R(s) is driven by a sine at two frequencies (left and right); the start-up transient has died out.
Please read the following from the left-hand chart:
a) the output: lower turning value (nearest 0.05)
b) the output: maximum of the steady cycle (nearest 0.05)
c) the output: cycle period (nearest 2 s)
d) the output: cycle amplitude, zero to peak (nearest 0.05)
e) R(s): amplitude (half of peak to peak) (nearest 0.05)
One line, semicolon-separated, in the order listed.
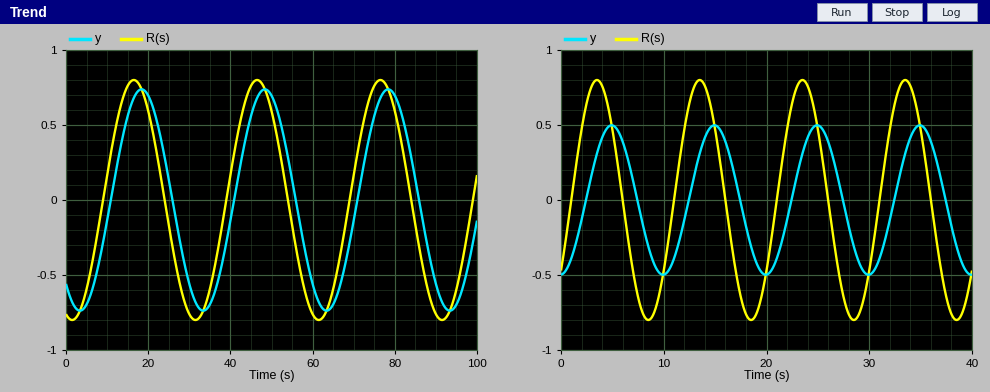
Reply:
-0.75; 0.75; 30 s; 0.75; 0.80
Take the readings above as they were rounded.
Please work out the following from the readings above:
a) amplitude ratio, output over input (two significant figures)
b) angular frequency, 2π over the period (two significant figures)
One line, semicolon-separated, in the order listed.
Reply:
0.94; 0.21 rad/s
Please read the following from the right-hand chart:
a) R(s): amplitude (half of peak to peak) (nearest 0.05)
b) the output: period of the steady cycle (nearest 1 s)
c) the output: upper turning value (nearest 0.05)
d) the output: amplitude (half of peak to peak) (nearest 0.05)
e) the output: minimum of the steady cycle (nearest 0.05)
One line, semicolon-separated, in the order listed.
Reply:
0.80; 10 s; 0.50; 0.50; -0.50
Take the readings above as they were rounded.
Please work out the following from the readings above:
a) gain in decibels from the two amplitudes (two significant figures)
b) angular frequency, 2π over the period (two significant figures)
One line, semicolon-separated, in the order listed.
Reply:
-4.1 dB; 0.63 rad/s
